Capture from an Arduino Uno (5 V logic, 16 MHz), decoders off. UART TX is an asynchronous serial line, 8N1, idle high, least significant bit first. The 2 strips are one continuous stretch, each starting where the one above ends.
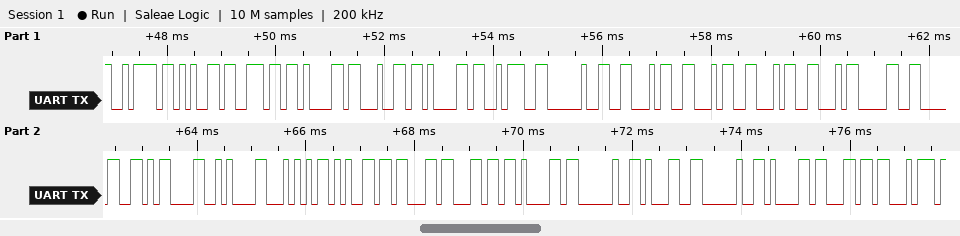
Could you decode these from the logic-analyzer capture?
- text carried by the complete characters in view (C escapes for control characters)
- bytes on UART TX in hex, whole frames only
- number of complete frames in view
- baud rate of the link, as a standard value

"zenada: FFFF00\r\nTecla 1 alt"
7A 65 6E 61 64 61 3A 20 46 46 46 46 30 30 0D 0A 54 65 63 6C 61 20 31 20 61 6C 74
27
9600 baud
